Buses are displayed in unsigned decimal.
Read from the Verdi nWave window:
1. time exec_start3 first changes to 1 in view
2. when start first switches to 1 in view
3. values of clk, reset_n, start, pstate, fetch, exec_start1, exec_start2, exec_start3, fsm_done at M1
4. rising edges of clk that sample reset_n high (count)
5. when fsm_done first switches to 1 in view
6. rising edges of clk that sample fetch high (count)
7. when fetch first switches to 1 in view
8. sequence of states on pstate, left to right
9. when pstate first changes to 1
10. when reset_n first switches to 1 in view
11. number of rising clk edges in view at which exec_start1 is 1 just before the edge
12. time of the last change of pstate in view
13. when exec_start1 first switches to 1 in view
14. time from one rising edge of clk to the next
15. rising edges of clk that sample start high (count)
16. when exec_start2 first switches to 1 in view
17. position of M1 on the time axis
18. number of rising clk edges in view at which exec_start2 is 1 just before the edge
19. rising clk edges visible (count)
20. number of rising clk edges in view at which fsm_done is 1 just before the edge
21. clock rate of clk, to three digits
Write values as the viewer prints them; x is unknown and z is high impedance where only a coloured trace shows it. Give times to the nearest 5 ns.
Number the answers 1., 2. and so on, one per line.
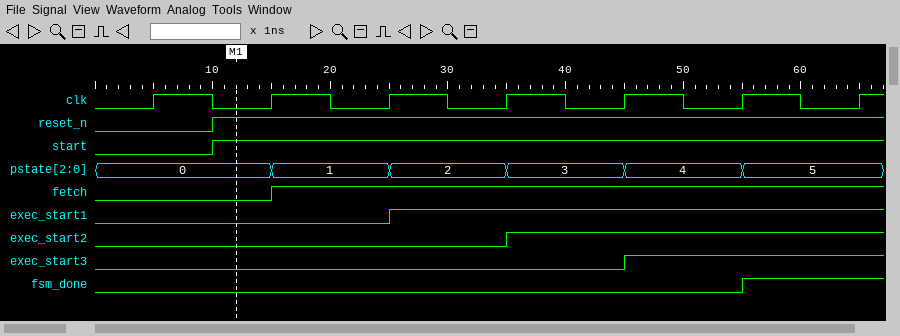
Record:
1. 45 ns
2. 10 ns
3. clk=0, reset_n=1, start=1, pstate=0, fetch=0, exec_start1=0, exec_start2=0, exec_start3=0, fsm_done=0
4. 6
5. 55 ns
6. 5
7. 15 ns
8. 0, 1, 2, 3, 4, 5
9. 15 ns
10. 10 ns
11. 4
12. 55 ns
13. 25 ns
14. 10 ns
15. 6
16. 35 ns
17. 10 ns
18. 3
19. 7
20. 1
21. 100 MHz
